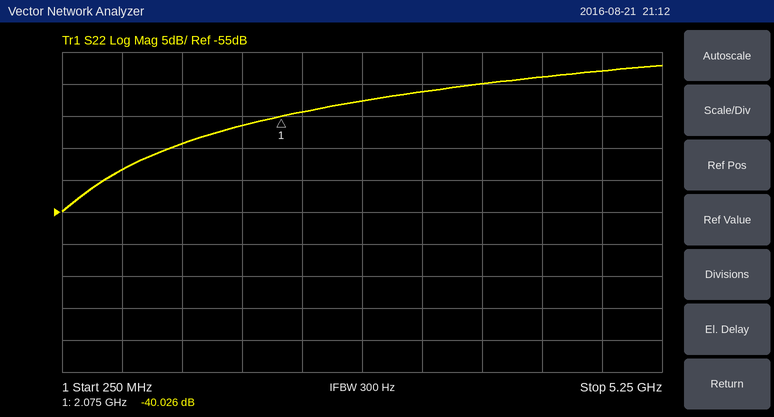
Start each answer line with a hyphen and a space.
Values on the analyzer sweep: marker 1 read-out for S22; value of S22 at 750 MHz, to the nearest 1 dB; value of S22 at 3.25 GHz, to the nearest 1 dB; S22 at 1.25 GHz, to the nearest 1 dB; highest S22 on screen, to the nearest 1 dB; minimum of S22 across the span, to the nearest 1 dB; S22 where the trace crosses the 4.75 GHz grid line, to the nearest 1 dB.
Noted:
- -40.026 dB
- -48 dB
- -36 dB
- -44 dB
- -32 dB
- -55 dB
- -33 dB
